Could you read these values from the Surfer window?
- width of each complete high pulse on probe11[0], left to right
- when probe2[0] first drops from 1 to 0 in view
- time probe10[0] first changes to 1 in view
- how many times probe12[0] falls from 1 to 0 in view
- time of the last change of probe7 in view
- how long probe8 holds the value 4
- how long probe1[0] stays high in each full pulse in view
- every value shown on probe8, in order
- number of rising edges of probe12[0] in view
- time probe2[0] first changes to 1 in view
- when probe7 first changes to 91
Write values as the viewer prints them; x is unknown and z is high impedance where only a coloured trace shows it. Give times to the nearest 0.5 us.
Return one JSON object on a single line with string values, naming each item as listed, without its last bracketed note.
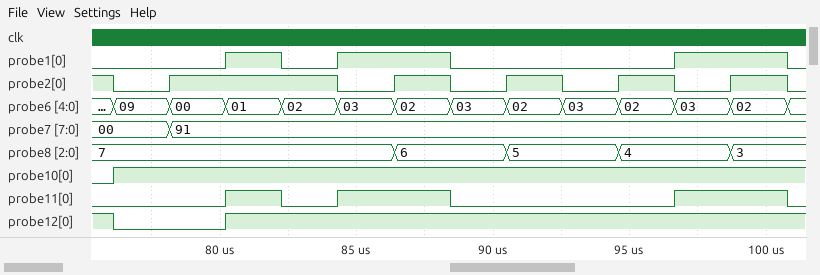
{"width of each complete high pulse on probe11[0], left to right": "2 us, 4 us, 4 us", "when probe2[0] first drops from 1 to 0 in view": "76 us", "time probe10[0] first changes to 1 in view": "76 us", "how many times probe12[0] falls from 1 to 0 in view": "1", "time of the last change of probe7 in view": "78 us", "how long probe8 holds the value 4": "4 us", "how long probe1[0] stays high in each full pulse in view": "2 us, 4 us, 4 us", "every value shown on probe8, in order": "7, 6, 5, 4, 3", "number of rising edges of probe12[0] in view": "1", "time probe2[0] first changes to 1 in view": "78 us", "when probe7 first changes to 91": "78 us"}
